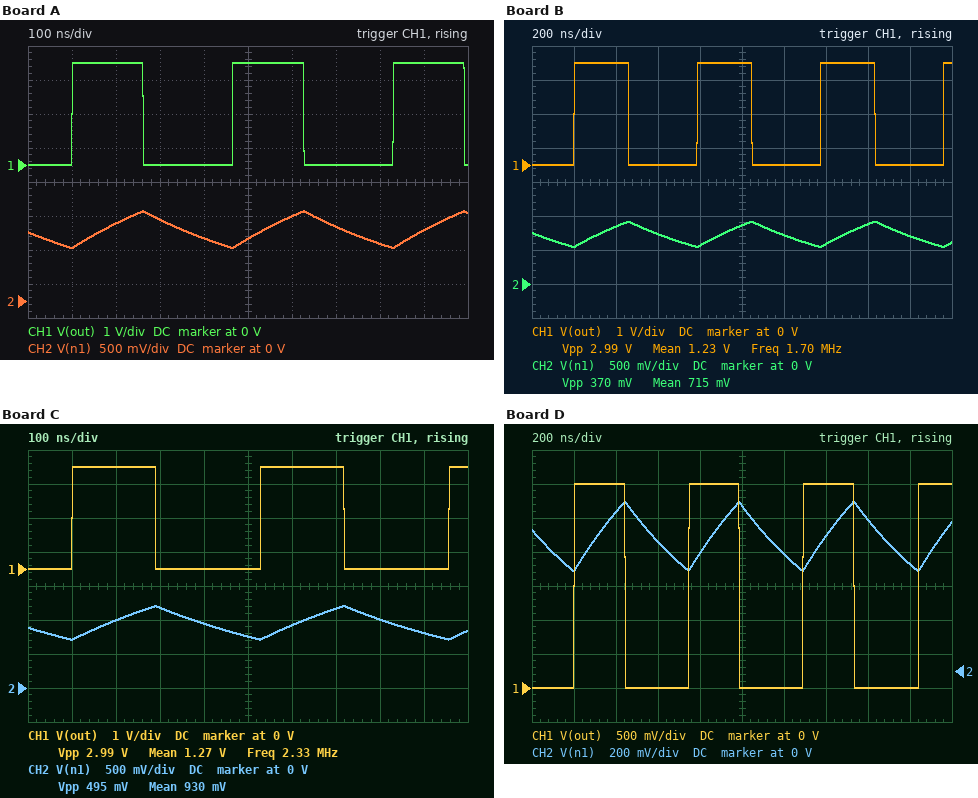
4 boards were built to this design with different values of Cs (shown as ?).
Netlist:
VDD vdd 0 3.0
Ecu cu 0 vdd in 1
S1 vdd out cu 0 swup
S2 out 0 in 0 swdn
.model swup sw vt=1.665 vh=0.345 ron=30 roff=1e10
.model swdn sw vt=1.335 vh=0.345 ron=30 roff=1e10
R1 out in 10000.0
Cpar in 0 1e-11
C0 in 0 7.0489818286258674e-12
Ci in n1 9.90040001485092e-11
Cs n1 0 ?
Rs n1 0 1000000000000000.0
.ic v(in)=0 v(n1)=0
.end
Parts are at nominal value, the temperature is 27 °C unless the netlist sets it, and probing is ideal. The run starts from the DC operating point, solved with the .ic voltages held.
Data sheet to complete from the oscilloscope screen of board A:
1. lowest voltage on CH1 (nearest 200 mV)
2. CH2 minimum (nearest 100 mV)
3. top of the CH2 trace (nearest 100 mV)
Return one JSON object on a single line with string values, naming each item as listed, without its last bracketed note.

{"lowest voltage on CH1": "0 V", "CH2 minimum": "800 mV", "top of the CH2 trace": "1.3 V"}
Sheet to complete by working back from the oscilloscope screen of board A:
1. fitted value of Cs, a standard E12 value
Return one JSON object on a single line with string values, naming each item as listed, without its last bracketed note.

{"fitted value of Cs, a standard E12 value": "27 pF"}
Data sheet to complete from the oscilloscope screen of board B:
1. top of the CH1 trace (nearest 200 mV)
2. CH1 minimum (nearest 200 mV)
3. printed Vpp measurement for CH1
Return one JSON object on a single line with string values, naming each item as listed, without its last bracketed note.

{"top of the CH1 trace": "3.0 V", "CH1 minimum": "0 V", "printed Vpp measurement for CH1": "2.99 V"}
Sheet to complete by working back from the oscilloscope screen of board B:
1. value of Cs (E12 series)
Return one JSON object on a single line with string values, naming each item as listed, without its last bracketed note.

{"value of Cs": "82 pF"}
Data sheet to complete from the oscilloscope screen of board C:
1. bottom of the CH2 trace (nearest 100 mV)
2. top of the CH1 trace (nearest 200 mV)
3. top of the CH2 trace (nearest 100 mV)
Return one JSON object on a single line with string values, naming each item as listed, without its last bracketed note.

{"bottom of the CH2 trace": "700 mV", "top of the CH1 trace": "3.0 V", "top of the CH2 trace": "1.2 V"}
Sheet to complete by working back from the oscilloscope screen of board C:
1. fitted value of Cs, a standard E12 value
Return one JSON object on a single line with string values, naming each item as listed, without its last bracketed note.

{"fitted value of Cs, a standard E12 value": "39 pF"}
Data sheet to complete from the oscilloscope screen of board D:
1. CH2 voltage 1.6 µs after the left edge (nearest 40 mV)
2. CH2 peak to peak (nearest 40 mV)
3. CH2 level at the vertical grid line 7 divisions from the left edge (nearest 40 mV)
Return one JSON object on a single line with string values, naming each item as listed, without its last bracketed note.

{"CH2 voltage 1.6 µs after the left edge": "880 mV", "CH2 peak to peak": "400 mV", "CH2 level at the vertical grid line 7 divisions from the left edge": "800 mV"}
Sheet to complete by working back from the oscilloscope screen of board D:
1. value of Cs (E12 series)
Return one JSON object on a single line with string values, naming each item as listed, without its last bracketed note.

{"value of Cs": "68 pF"}
